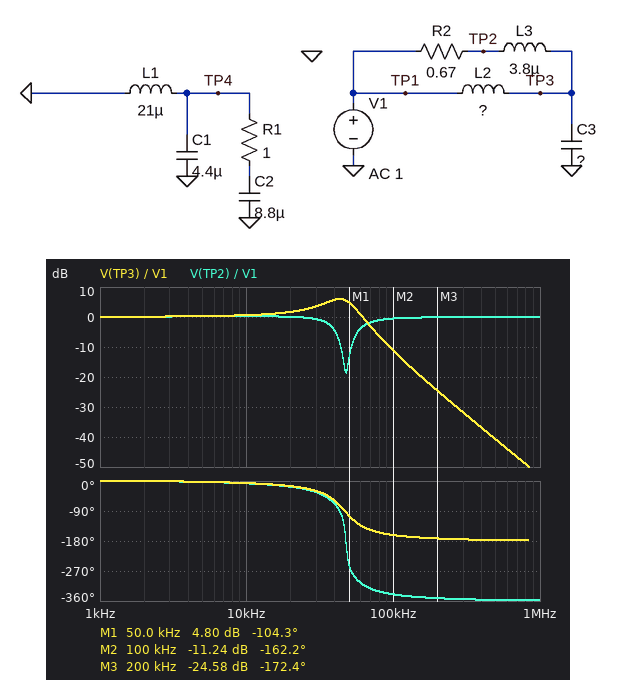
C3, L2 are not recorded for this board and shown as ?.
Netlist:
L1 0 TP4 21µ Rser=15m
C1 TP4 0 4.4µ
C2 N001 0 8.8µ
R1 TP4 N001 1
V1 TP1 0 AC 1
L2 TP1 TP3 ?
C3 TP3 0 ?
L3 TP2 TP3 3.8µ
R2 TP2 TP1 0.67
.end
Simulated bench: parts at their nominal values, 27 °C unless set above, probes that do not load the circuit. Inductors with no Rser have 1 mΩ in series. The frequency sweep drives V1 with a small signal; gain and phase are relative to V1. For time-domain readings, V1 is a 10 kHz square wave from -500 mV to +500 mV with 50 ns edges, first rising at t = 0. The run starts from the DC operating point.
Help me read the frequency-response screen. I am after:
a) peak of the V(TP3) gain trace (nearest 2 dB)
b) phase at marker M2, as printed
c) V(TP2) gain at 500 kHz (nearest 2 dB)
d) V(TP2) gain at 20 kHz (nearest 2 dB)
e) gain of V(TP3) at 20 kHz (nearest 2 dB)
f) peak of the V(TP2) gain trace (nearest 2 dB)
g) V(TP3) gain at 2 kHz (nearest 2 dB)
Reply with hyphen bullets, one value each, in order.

- 6 dB
- -162.2 deg
- 0 dB
- 0 dB
- 2 dB
- 0 dB
- 0 dB
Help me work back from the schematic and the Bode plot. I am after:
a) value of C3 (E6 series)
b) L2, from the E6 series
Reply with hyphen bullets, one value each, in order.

- 3.3 µF
- 33 µH
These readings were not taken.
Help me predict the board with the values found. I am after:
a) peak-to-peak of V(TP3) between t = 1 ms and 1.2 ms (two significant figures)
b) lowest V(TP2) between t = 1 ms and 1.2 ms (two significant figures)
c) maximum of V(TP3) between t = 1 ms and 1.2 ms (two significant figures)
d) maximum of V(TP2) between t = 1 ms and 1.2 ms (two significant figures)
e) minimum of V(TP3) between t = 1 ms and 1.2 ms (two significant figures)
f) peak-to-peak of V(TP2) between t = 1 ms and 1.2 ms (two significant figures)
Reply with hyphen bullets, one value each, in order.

- 1.9 V
- -700 mV
- 950 mV
- 700 mV
- -950 mV
- 1.4 V
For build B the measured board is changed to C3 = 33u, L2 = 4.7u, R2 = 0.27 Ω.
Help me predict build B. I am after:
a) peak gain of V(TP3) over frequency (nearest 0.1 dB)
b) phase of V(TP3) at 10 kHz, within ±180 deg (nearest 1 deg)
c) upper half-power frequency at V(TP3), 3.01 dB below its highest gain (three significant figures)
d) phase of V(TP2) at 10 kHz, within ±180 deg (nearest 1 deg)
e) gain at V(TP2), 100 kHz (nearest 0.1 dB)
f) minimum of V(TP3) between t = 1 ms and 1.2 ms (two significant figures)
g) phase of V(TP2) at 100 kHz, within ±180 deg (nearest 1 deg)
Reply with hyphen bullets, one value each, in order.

- 10.8 dB
- -12 deg
- 20.5 kHz
- -20 deg
- -0.1 dB
- -1.0 V
- 7 deg
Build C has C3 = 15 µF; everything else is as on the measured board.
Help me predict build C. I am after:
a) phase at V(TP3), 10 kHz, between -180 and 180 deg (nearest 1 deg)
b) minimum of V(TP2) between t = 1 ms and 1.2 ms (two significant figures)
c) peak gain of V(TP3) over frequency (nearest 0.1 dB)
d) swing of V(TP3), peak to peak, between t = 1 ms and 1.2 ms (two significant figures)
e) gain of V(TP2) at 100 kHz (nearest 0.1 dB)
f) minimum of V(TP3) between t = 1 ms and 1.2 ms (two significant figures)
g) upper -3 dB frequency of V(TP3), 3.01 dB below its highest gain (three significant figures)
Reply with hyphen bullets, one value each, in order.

- -35 deg
- -670 mV
- 1.8 dB
- 1.4 V
- -0.4 dB
- -710 mV
- 22.6 kHz
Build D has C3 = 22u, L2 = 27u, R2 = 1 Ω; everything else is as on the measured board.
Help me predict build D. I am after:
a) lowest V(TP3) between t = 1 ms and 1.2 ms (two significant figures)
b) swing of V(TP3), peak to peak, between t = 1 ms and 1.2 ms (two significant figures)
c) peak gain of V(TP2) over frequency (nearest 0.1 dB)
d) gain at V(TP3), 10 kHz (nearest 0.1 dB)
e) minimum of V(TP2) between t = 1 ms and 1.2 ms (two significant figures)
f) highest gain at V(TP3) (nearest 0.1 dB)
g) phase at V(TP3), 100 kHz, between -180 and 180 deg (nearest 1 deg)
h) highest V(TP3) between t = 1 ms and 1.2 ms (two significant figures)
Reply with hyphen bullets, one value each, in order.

- -750 mV
- 1.5 V
- 2.8 dB
- 1.1 dB
- -710 mV
- 3.3 dB
- -160 deg
- 750 mV
